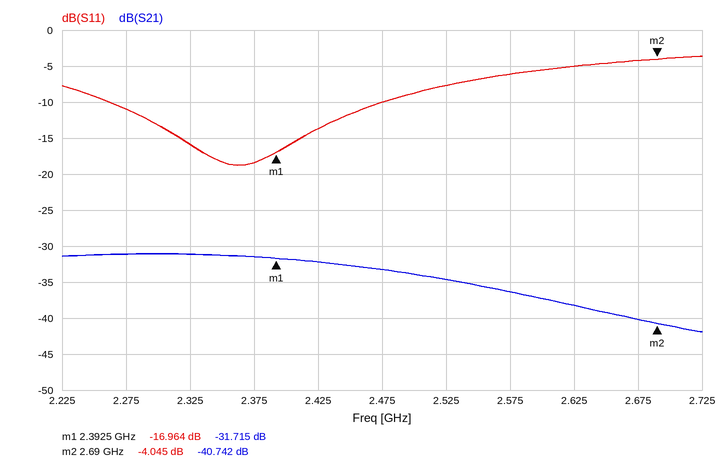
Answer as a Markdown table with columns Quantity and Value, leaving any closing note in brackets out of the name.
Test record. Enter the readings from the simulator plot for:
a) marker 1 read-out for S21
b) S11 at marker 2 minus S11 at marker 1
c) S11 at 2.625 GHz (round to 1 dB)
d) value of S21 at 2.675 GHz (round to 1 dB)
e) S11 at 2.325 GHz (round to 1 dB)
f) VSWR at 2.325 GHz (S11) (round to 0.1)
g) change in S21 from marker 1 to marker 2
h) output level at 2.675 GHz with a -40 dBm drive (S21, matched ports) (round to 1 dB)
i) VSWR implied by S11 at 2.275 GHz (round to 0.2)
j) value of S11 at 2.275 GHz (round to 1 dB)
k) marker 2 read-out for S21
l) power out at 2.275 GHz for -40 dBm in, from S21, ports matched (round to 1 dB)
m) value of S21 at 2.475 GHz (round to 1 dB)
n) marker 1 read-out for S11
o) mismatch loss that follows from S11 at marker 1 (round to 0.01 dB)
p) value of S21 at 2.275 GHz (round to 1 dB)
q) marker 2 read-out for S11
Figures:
| Quantity | Value |
|---|---|
| marker 1 read-out for S21 | -31.715 dB |
| S11 at marker 2 minus S11 at marker 1 | 12.919 dB |
| S11 at 2.625 GHz | -5 dB |
| value of S21 at 2.675 GHz | -40 dB |
| S11 at 2.325 GHz | -16 dB |
| VSWR at 2.325 GHz (S11) | 1.4 |
| change in S21 from marker 1 to marker 2 | -9.027 dB |
| output level at 2.675 GHz with a -40 dBm drive (S21, matched ports) | -80 dBm |
| VSWR implied by S11 at 2.275 GHz | 1.8 |
| value of S11 at 2.275 GHz | -11 dB |
| marker 2 read-out for S21 | -40.742 dB |
| power out at 2.275 GHz for -40 dBm in, from S21, ports matched | -71 dBm |
| value of S21 at 2.475 GHz | -33 dB |
| marker 1 read-out for S11 | -16.964 dB |
| mismatch loss that follows from S11 at marker 1 | 0.09 dB |
| value of S21 at 2.275 GHz | -31 dB |
| marker 2 read-out for S11 | -4.045 dB |
